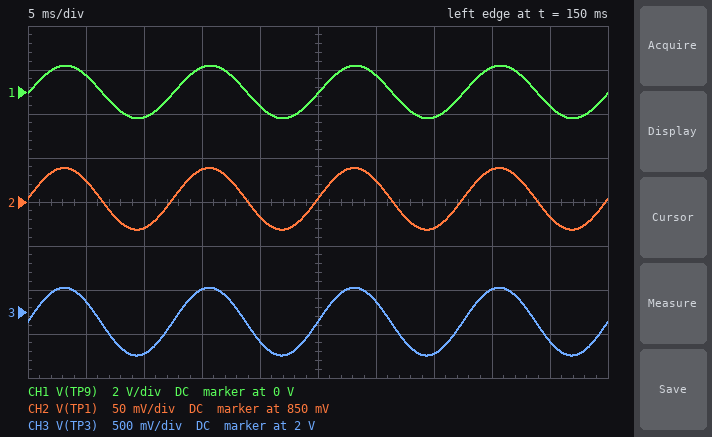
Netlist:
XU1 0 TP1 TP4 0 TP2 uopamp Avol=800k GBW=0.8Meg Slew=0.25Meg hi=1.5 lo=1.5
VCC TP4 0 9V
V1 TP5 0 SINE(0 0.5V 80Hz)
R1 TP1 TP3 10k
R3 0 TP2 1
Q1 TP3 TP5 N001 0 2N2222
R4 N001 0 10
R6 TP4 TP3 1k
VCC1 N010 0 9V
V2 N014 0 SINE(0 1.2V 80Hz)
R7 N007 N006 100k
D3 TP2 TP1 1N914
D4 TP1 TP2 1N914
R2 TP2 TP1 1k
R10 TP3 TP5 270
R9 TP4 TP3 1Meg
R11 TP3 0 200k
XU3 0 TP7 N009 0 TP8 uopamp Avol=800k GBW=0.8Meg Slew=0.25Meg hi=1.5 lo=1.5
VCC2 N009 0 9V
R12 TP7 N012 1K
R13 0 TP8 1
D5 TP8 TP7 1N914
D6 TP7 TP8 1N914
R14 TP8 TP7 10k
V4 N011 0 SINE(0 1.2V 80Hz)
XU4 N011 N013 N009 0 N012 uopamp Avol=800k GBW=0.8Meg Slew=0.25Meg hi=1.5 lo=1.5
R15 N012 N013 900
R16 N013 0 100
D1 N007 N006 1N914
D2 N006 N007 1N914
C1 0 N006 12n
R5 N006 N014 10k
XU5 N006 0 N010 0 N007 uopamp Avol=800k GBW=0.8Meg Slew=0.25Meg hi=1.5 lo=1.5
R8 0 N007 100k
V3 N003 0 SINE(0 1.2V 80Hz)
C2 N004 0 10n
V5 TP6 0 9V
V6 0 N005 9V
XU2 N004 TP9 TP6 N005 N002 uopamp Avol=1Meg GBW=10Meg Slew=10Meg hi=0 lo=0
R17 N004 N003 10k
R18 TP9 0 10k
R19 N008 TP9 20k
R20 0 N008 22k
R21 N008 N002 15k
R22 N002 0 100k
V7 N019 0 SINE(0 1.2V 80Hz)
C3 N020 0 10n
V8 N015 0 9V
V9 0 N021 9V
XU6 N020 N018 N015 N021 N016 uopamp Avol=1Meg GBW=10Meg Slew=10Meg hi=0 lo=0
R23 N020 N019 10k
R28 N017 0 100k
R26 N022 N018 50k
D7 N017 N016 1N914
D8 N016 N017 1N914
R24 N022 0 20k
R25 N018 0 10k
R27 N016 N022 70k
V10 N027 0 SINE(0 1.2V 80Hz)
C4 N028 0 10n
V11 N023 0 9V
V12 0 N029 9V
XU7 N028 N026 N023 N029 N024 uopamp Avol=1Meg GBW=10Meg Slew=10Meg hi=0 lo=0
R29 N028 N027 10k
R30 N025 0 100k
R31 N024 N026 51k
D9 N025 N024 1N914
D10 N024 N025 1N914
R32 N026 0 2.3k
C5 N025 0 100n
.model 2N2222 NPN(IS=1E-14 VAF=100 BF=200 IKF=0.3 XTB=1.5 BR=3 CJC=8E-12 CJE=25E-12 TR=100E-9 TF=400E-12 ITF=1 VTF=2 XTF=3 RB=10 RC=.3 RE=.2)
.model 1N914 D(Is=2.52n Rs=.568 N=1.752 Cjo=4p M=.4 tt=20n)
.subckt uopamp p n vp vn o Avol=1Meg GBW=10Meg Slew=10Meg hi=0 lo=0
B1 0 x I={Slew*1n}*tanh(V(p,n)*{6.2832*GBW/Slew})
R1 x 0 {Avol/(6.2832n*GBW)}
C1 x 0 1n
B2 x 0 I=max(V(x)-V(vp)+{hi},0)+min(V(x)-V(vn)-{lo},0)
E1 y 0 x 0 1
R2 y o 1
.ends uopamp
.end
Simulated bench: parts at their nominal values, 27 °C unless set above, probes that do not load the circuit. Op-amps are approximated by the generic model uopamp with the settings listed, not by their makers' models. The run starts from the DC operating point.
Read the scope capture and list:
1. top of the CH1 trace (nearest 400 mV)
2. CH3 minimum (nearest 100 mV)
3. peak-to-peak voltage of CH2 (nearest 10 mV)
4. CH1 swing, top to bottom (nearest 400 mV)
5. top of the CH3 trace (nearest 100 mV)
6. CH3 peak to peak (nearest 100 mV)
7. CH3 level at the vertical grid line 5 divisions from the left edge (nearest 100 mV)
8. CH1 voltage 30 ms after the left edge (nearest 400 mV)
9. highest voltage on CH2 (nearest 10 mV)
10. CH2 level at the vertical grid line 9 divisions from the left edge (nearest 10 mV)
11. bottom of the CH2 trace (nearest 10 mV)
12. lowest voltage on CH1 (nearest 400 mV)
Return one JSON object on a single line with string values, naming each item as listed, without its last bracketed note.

{"top of the CH1 trace": "1.2 V", "CH3 minimum": "1.5 V", "peak-to-peak voltage of CH2": "70 mV", "CH1 swing, top to bottom": "2.4 V", "top of the CH3 trace": "2.3 V", "CH3 peak to peak": "800 mV", "CH3 level at the vertical grid line 5 divisions from the left edge": "1.9 V", "CH1 voltage 30 ms after the left edge": "800 mV", "highest voltage on CH2": "890 mV", "CH2 level at the vertical grid line 9 divisions from the left edge": "830 mV", "bottom of the CH2 trace": "820 mV", "lowest voltage on CH1": "-1.2 V"}
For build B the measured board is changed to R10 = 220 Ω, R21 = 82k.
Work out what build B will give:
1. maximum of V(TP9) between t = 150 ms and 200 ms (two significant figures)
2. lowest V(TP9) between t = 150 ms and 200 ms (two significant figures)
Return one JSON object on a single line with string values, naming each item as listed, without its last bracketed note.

{"maximum of V(TP9) between t = 150 ms and 200 ms": "400 mV", "lowest V(TP9) between t = 150 ms and 200 ms": "-400 mV"}
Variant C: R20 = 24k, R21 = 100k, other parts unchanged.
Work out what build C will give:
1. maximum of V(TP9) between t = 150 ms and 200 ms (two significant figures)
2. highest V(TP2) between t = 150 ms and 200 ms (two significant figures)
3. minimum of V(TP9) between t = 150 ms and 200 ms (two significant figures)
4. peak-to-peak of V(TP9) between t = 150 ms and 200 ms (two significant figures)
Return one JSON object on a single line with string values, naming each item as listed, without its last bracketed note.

{"maximum of V(TP9) between t = 150 ms and 200 ms": "350 mV", "highest V(TP2) between t = 150 ms and 200 ms": "750 mV", "minimum of V(TP9) between t = 150 ms and 200 ms": "-350 mV", "peak-to-peak of V(TP9) between t = 150 ms and 200 ms": "710 mV"}
